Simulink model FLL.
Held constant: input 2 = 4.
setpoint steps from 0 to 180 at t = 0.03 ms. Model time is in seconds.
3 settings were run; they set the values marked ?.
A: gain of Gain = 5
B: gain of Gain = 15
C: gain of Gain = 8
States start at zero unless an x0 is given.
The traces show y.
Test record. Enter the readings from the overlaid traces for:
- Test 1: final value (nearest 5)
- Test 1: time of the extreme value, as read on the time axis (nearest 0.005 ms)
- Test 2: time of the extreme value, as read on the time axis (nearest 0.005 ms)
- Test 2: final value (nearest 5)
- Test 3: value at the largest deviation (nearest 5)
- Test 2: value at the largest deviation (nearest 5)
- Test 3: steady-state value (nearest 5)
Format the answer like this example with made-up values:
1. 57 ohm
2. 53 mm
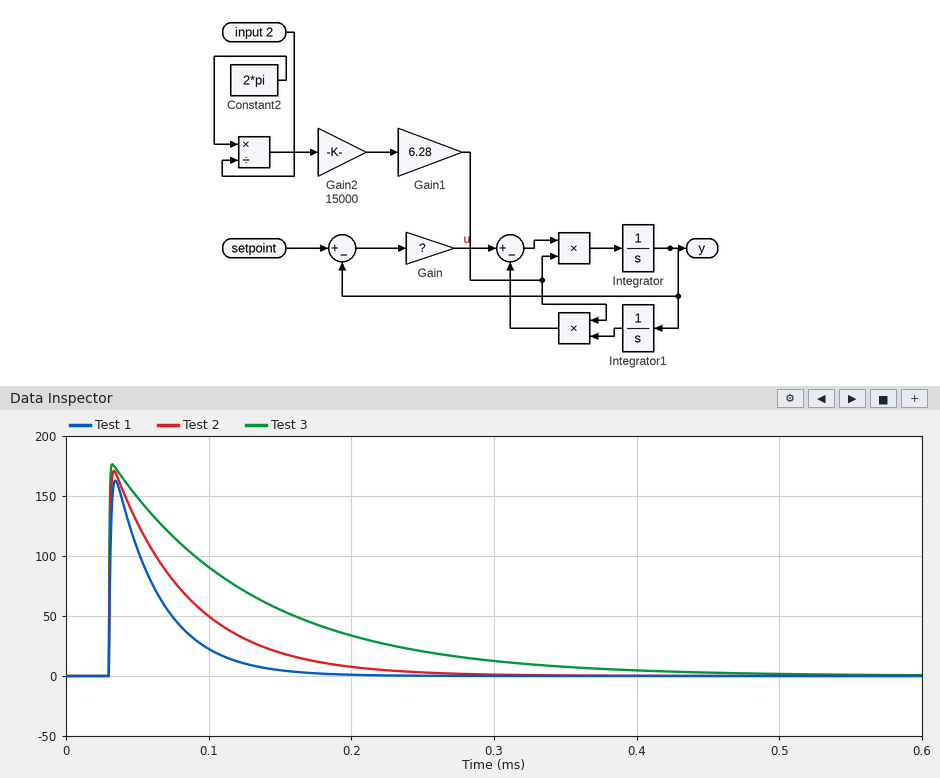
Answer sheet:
1. 0
2. 0.035 ms
3. 0.035 ms
4. 0
5. 175
6. 170
7. 0
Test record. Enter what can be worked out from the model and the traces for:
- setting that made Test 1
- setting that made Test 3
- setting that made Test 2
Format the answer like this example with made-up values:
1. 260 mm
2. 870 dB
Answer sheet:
1. A
2. B
3. C
